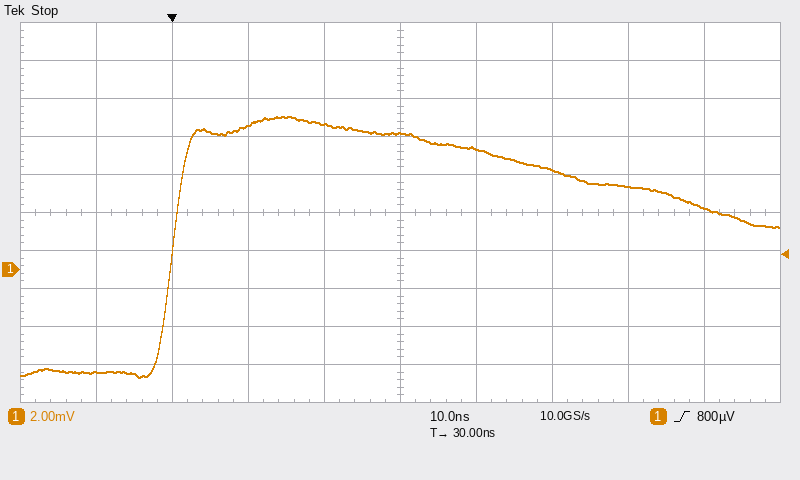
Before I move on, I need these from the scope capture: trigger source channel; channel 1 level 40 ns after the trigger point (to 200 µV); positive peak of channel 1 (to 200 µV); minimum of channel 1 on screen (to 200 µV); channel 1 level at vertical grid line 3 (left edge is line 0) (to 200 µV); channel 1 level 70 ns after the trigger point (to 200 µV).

channel 1
6.4 mV
8.0 mV
-5.6 mV
7.6 mV
3.2 mV
